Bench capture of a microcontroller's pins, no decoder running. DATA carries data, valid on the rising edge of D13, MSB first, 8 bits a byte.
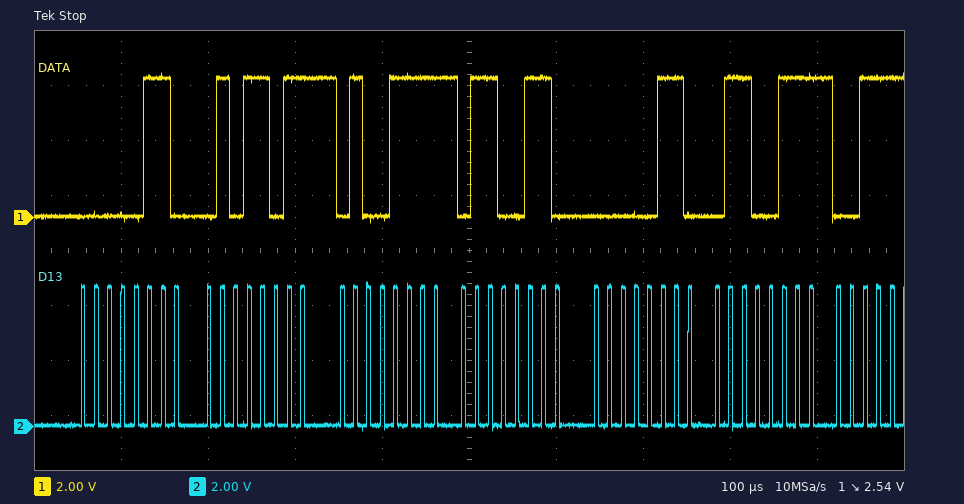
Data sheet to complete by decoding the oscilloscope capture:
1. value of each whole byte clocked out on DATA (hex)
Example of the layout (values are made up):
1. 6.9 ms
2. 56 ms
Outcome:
1. 06 5B 4F 66 06 67
